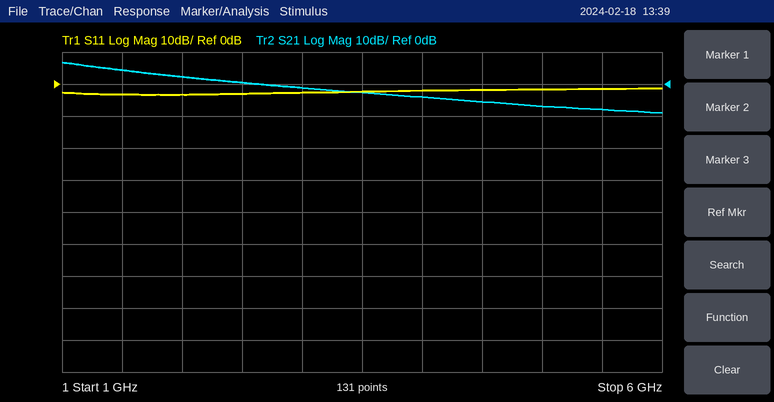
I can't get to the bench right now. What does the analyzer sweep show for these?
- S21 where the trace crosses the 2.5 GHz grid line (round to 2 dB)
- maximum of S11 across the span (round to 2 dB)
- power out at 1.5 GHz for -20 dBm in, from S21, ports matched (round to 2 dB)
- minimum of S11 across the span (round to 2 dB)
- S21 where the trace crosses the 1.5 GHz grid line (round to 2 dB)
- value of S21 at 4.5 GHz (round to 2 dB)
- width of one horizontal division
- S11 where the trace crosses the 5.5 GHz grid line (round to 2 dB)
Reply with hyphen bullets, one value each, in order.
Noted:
- 0 dB
- -2 dB
- -16 dBm
- -4 dB
- 4 dB
- -6 dB
- 500 MHz
- -2 dB
